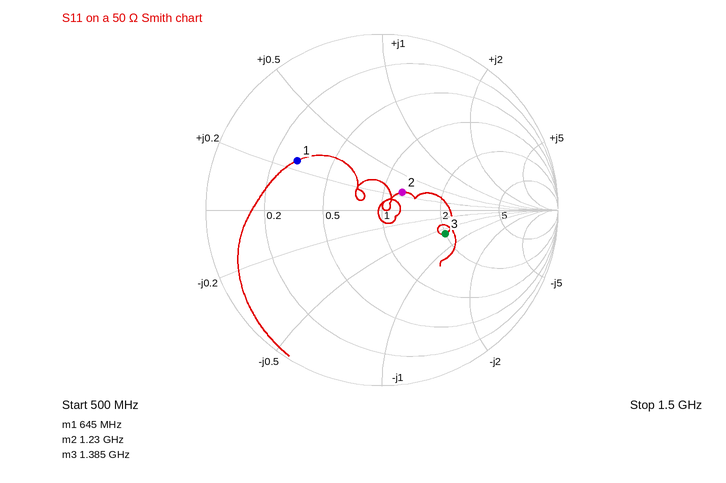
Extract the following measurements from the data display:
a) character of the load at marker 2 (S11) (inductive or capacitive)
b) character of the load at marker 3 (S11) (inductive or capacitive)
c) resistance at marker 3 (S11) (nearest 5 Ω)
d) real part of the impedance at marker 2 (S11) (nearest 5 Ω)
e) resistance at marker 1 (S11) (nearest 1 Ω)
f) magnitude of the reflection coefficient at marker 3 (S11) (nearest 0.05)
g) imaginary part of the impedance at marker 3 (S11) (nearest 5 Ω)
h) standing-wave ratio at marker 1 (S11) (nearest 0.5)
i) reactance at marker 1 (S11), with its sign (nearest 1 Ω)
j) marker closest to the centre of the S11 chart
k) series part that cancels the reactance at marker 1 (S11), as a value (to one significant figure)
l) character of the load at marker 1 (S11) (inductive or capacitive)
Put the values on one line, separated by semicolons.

inductive; capacitive; 100 Ω; 60 Ω; 15 Ω; 0.40; -30 Ω; 3.5; +12 Ω; marker 2; 20 pF; inductive
